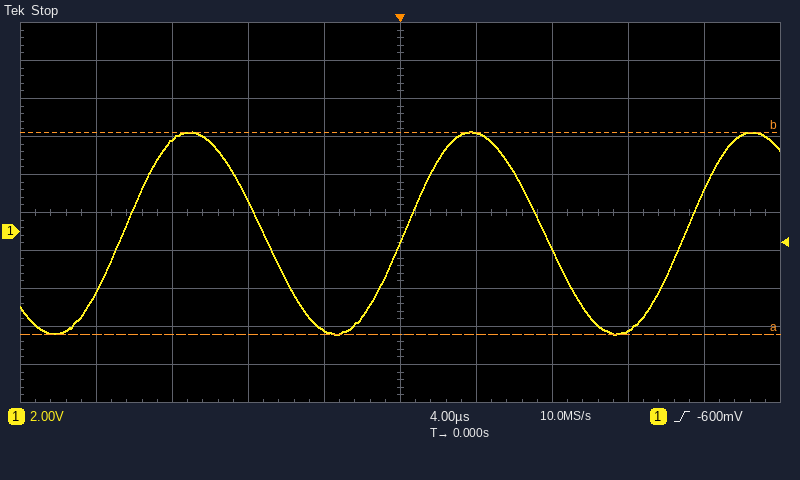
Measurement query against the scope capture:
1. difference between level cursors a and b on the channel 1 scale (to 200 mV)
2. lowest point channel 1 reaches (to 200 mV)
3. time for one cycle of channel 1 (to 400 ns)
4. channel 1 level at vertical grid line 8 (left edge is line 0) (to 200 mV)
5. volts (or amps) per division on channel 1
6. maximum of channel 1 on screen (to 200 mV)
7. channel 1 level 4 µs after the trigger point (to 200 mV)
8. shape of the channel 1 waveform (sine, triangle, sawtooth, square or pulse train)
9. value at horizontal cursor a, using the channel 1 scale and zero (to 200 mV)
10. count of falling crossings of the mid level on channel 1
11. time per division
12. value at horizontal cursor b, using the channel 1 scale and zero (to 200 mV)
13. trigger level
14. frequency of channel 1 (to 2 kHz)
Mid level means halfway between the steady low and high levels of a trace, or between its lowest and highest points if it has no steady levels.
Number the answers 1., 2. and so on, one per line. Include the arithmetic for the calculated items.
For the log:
1. 10.6 V
2. -5.4 V
3. 14.8 µs
4. -5.2 V
5. 2 V
6. 5.2 V
7. 5.2 V
8. sine
9. -5.4 V
10. 2
11. 4 µs
12. 5.2 V
13. -600 mV
14. 1 / 14.8 µs ≈ 68 kHz
